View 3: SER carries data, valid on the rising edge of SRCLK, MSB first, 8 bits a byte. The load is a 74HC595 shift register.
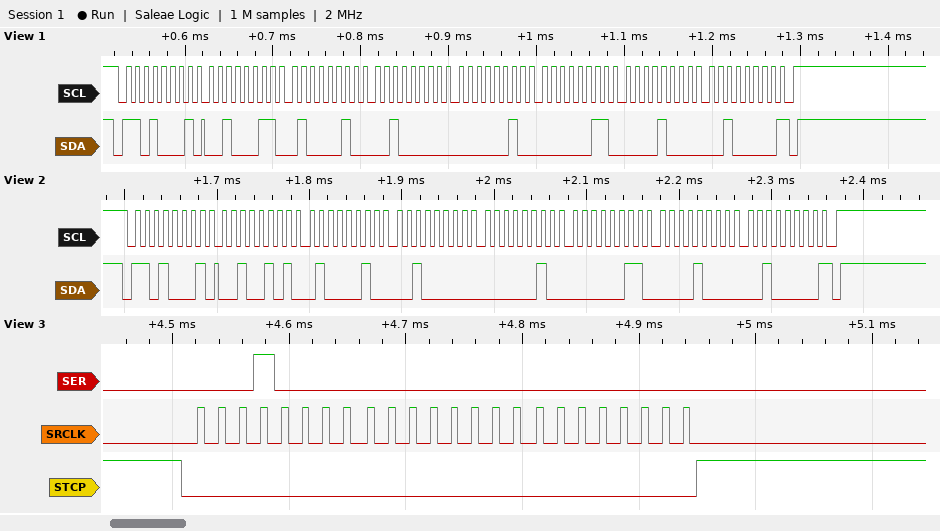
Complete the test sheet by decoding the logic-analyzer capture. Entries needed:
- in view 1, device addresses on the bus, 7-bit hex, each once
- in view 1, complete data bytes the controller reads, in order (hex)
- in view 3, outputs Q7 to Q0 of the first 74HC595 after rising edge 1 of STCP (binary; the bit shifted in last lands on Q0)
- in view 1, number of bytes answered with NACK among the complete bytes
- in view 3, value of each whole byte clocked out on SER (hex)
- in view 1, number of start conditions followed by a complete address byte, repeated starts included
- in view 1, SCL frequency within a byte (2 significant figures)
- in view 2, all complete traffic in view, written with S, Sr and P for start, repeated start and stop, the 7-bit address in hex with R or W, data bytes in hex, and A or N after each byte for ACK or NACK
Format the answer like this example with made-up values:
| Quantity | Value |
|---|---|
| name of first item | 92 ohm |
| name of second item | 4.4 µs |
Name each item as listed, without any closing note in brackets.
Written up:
| Quantity | Value |
|---|---|
| in view 1, device addresses on the bus, 7-bit hex, each once | 0x68 |
| in view 1, complete data bytes the controller reads, in order | 23 42 20 02 03 08 20 |
| in view 3, outputs Q7 to Q0 of the first 74HC595 after rising edge 1 of STCP | 00000000 |
| in view 1, number of bytes answered with NACK among the complete bytes | 1 |
| in view 3, value of each whole byte clocked out on SER | 10 00 00 |
| in view 1, number of start conditions followed by a complete address byte, repeated starts included | 1 |
| in view 1, SCL frequency within a byte | 100 kHz |
| in view 2, all complete traffic in view, written with S, Sr and P for start, repeated start and stop, the 7-bit address in hex with R or W, data bytes in hex, and A or N after each byte for ACK or NACK | S 68R A 25 A 42 A 20 A 02 A 03 A 08 A 20 N P |
